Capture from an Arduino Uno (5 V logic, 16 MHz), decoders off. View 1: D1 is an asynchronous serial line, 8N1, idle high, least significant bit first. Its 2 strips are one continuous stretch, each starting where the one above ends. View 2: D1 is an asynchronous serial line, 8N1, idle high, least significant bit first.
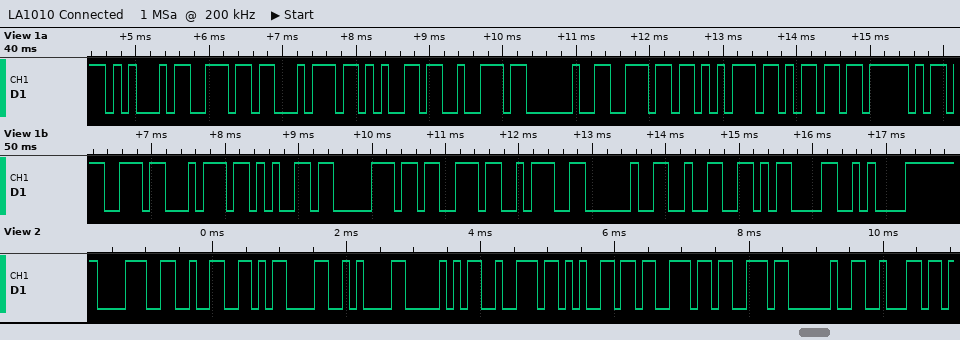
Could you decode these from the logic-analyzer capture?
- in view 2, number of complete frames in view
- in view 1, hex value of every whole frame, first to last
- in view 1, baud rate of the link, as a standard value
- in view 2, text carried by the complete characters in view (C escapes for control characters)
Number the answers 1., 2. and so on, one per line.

1. 11
2. 45 6E 74 65 72 20 6E 75 6D 5F 73 74 65 70 73 3A 20 32 0D 0A
3. 9600 baud
4. "82\r\nPress b"
